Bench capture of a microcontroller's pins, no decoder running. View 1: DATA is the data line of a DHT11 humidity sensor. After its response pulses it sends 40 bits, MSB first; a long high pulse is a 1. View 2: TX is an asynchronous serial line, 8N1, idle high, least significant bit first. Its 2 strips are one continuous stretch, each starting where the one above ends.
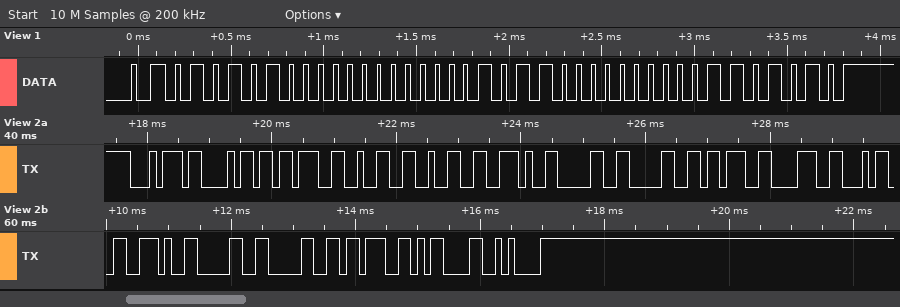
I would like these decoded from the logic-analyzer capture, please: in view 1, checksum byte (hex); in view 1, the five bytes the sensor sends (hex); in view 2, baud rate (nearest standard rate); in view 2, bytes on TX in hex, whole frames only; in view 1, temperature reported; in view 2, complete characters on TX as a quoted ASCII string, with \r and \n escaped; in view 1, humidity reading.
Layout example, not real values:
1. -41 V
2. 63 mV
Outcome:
1. 0x6A
2. 54 00 16 00 6A
3. 9600 baud
4. 0x74 0x68 0x3B 0x32 0x32 0x2E 0x30 0x30 0x3B 0x38 0x34 0x2E 0x30 0x30 0x3B 0x0D 0x0A
5. 22.0 °C
6. "th;22.00;84.00;\r\n"
7. 84 %
